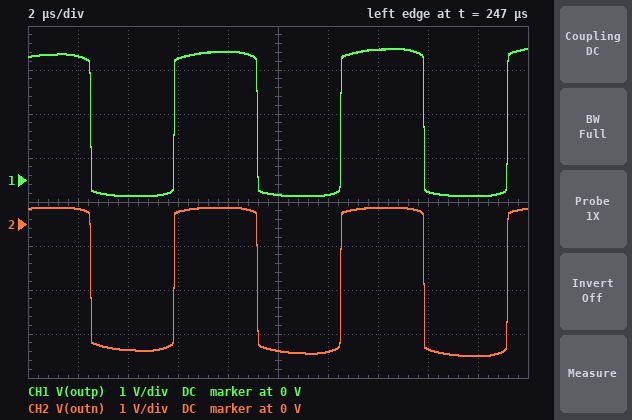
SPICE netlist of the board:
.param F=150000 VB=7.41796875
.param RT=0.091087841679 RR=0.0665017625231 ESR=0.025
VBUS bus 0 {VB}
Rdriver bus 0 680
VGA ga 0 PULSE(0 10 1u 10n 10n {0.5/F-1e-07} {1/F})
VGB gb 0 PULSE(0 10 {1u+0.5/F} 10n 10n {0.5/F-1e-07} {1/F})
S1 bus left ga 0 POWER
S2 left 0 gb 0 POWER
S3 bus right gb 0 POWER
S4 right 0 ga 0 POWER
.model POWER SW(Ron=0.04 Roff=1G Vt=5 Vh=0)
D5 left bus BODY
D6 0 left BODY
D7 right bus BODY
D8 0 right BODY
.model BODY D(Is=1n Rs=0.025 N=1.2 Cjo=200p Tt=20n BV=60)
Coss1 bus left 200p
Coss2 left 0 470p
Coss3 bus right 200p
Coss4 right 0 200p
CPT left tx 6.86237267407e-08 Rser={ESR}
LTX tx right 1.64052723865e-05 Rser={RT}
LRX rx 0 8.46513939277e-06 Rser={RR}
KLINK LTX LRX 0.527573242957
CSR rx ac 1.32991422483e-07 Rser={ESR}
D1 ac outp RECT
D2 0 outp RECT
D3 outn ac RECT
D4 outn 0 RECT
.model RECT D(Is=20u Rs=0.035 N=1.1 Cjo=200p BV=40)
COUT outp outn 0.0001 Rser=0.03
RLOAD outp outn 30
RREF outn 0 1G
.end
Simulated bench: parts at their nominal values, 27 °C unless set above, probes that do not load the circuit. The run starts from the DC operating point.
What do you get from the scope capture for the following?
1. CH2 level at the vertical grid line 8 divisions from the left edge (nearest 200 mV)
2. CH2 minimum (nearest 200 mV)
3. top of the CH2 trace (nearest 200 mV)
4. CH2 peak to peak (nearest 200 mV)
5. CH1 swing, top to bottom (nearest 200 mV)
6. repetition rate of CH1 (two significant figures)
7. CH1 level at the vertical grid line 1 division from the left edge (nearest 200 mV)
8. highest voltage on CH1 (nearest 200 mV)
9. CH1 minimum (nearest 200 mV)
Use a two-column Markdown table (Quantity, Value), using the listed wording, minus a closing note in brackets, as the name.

| Quantity | Value |
|---|---|
| CH2 level at the vertical grid line 8 divisions from the left edge | -2.8 V |
| CH2 minimum | -3.0 V |
| top of the CH2 trace | 400 mV |
| CH2 peak to peak | 3.4 V |
| CH1 swing, top to bottom | 3.4 V |
| repetition rate of CH1 | 150 kHz |
| CH1 level at the vertical grid line 1 division from the left edge | 2.8 V |
| highest voltage on CH1 | 3.0 V |
| CH1 minimum | -400 mV |
